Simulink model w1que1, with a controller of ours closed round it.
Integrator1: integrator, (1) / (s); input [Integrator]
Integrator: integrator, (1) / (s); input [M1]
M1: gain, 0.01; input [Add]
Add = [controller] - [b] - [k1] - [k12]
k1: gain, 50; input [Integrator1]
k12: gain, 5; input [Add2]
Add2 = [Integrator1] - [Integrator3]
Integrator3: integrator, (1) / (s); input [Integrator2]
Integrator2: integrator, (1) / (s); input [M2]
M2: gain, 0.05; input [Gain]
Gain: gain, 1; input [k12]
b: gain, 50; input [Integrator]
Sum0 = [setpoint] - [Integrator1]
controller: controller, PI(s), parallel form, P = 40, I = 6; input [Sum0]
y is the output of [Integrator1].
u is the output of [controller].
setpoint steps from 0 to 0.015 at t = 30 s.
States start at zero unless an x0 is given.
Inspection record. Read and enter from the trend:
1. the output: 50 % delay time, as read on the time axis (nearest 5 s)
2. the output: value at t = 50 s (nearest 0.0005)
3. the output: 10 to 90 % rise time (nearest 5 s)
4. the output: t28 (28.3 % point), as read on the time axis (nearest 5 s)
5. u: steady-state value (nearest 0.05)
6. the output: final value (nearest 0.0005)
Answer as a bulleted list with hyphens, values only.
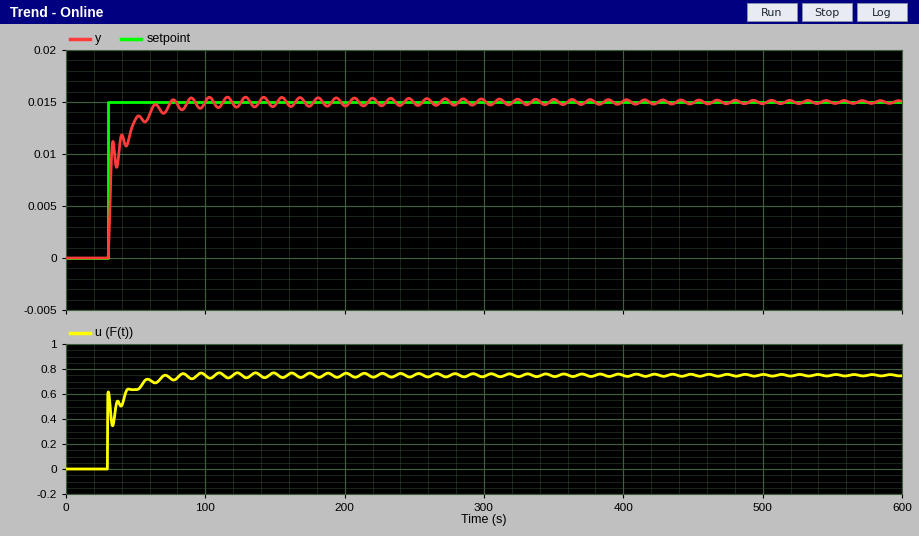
- 30 s
- 0.0135
- 20 s
- 30 s
- 0.75
- 0.0150
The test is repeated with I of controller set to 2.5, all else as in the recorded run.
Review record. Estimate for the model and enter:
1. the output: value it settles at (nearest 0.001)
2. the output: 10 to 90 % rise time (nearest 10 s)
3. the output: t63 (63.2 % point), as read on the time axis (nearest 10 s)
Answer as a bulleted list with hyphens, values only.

- 0.015
- 60 s
- 30 s
